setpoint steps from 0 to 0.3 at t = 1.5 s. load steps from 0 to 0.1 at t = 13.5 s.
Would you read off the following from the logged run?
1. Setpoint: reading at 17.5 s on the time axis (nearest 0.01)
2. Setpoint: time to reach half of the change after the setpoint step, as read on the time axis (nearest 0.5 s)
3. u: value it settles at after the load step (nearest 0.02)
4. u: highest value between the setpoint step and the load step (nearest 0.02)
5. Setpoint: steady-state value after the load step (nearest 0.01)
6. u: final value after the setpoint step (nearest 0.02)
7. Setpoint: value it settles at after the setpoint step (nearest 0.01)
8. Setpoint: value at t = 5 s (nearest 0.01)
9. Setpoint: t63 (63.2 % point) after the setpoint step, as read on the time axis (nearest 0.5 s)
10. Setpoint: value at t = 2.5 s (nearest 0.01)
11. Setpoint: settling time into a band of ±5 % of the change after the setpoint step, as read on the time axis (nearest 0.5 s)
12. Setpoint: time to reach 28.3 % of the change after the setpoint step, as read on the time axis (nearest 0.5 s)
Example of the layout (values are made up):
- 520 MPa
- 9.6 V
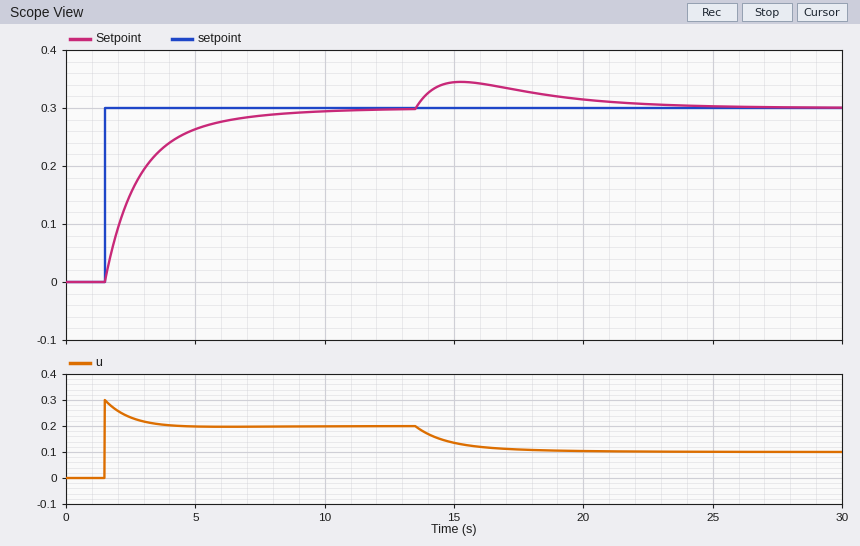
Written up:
- 0.33
- 2.5 s
- 0.10
- 0.30
- 0.30
- 0.20
- 0.30
- 0.26
- 3.0 s
- 0.15
- 7.0 s
- 2.0 s
